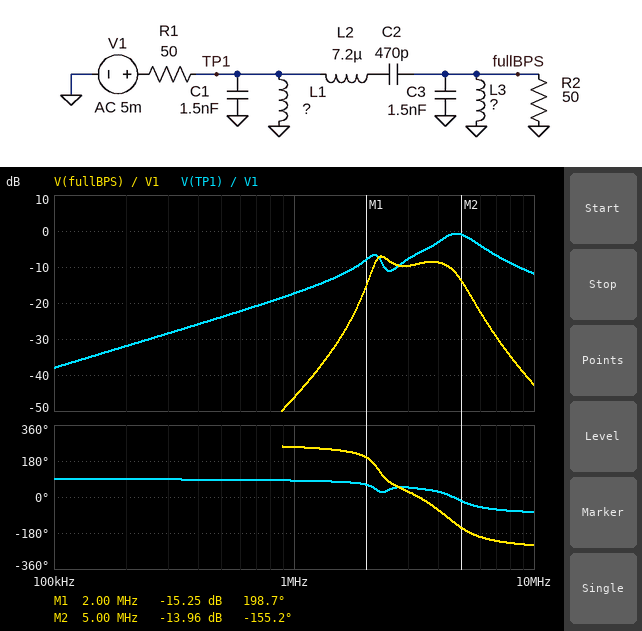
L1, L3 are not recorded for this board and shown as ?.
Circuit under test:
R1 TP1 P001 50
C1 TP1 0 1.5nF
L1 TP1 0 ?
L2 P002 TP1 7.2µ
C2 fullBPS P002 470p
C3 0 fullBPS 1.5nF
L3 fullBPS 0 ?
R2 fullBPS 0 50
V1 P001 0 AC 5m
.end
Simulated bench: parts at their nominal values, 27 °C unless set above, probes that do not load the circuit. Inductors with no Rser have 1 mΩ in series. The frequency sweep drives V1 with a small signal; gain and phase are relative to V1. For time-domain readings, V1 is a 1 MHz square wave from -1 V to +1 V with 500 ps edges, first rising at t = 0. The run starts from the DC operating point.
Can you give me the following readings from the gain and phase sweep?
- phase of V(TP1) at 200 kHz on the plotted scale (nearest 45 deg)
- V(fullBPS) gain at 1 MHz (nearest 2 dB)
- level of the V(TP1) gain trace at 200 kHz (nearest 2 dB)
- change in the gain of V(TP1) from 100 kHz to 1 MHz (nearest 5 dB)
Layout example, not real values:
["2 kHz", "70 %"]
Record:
["90 deg", "-46 dB", "-32 dB", "20 dB"]
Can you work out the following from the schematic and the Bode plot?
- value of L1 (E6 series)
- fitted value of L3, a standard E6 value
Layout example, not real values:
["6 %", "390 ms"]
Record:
["1 µH", "1.5 µH"]
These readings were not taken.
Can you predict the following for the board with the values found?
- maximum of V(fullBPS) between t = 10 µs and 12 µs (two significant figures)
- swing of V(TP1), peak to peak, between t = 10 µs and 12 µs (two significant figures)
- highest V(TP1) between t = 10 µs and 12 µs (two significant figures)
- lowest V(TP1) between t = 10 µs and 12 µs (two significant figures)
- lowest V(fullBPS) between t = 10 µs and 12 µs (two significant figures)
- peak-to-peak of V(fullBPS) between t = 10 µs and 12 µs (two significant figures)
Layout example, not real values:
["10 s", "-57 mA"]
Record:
["190 mV", "1.4 V", "680 mV", "-680 mV", "-190 mV", "380 mV"]
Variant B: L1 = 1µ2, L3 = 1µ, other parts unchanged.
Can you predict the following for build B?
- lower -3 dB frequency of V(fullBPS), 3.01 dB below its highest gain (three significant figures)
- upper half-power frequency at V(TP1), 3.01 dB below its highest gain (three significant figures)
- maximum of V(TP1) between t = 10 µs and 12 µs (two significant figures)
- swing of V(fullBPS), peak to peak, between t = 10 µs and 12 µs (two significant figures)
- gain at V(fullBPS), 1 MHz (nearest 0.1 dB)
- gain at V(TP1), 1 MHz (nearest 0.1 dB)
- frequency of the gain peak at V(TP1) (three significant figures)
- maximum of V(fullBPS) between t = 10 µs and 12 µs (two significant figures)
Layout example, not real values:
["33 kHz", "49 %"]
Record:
["2.20 MHz", "5.80 MHz", "680 mV", "350 mV", "-48.4 dB", "-15.7 dB", "4.37 MHz", "180 mV"]
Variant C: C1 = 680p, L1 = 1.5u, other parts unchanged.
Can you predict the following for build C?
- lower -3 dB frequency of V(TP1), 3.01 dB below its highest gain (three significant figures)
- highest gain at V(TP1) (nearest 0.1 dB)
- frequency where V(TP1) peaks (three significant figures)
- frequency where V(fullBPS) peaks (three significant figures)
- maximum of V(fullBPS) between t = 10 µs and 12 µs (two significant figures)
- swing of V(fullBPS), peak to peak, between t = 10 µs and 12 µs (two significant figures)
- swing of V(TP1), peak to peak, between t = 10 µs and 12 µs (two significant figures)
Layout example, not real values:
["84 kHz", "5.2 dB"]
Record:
["4.26 MHz", "-0.2 dB", "5.79 MHz", "2.28 MHz", "200 mV", "390 mV", "2.0 V"]
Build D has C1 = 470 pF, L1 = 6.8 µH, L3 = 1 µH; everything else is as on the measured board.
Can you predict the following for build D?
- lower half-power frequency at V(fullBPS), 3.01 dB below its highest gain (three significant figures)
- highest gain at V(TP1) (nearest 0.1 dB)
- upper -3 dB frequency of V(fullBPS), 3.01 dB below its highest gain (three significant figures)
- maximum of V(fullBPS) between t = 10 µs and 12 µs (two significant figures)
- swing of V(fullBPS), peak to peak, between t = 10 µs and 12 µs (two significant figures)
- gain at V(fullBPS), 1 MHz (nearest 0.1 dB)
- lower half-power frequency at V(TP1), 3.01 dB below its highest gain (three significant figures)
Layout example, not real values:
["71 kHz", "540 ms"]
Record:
["2.16 MHz", "-0.1 dB", "4.94 MHz", "240 mV", "480 mV", "-35.1 dB", "897 kHz"]
